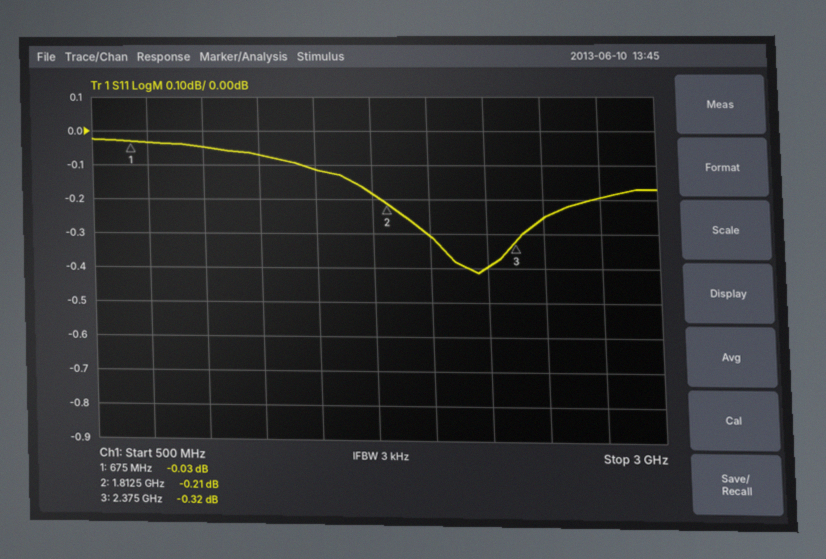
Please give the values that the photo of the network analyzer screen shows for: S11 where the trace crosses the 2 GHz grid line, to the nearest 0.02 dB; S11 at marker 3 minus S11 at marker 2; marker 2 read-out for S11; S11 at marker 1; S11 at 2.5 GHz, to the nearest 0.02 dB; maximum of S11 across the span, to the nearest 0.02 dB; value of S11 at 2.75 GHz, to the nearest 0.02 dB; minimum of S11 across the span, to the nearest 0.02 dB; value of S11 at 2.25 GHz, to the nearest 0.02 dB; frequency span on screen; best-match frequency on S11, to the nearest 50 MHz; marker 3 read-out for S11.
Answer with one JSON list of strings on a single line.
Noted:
["-0.30 dB", "-0.11 dB", "-0.21 dB", "-0.03 dB", "-0.26 dB", "-0.02 dB", "-0.20 dB", "-0.42 dB", "-0.40 dB", "2.5 GHz", "2.20 GHz", "-0.32 dB"]
